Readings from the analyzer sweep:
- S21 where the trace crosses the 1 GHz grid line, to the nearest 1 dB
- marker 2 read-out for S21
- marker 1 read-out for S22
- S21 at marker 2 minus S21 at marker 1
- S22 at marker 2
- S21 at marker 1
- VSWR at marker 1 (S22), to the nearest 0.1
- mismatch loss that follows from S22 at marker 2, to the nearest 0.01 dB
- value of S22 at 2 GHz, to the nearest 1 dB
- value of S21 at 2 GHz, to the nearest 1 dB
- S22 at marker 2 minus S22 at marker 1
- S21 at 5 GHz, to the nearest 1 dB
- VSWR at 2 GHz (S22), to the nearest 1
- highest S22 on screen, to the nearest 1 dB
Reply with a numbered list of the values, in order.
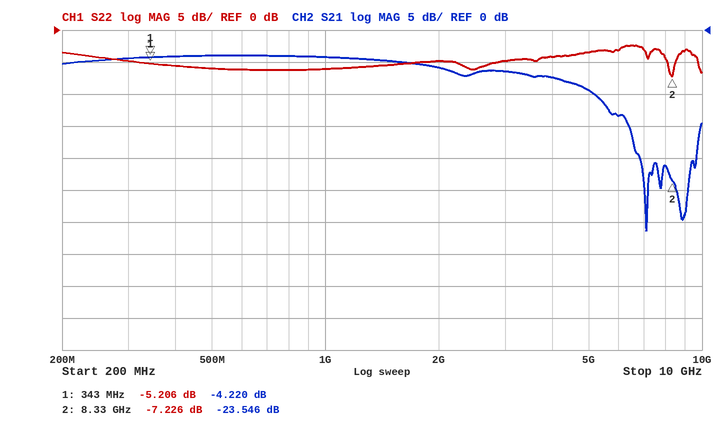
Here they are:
1. -4 dB
2. -23.546 dB
3. -5.206 dB
4. -19.326 dB
5. -7.226 dB
6. -4.220 dB
7. 3.4
8. 0.91 dB
9. -5 dB
10. -6 dB
11. -2.020 dB
12. -9 dB
13. 4
14. -2 dB
